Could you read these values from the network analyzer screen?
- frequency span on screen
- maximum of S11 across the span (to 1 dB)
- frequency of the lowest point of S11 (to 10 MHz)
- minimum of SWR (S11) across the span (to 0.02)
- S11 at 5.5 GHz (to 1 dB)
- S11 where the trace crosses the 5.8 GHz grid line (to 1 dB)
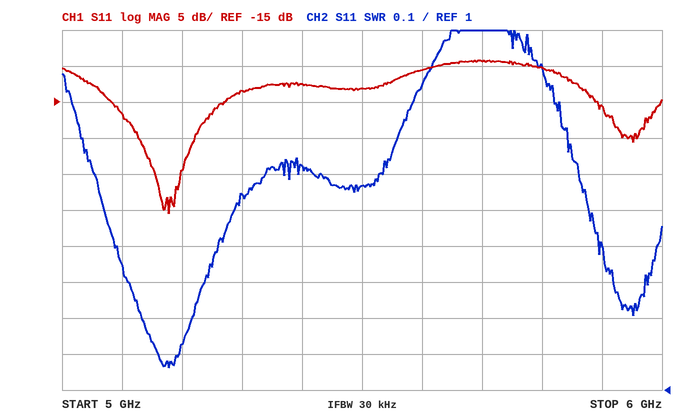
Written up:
1 GHz
-9 dB
5.18 GHz
1.06
-13 dB
-10 dB
